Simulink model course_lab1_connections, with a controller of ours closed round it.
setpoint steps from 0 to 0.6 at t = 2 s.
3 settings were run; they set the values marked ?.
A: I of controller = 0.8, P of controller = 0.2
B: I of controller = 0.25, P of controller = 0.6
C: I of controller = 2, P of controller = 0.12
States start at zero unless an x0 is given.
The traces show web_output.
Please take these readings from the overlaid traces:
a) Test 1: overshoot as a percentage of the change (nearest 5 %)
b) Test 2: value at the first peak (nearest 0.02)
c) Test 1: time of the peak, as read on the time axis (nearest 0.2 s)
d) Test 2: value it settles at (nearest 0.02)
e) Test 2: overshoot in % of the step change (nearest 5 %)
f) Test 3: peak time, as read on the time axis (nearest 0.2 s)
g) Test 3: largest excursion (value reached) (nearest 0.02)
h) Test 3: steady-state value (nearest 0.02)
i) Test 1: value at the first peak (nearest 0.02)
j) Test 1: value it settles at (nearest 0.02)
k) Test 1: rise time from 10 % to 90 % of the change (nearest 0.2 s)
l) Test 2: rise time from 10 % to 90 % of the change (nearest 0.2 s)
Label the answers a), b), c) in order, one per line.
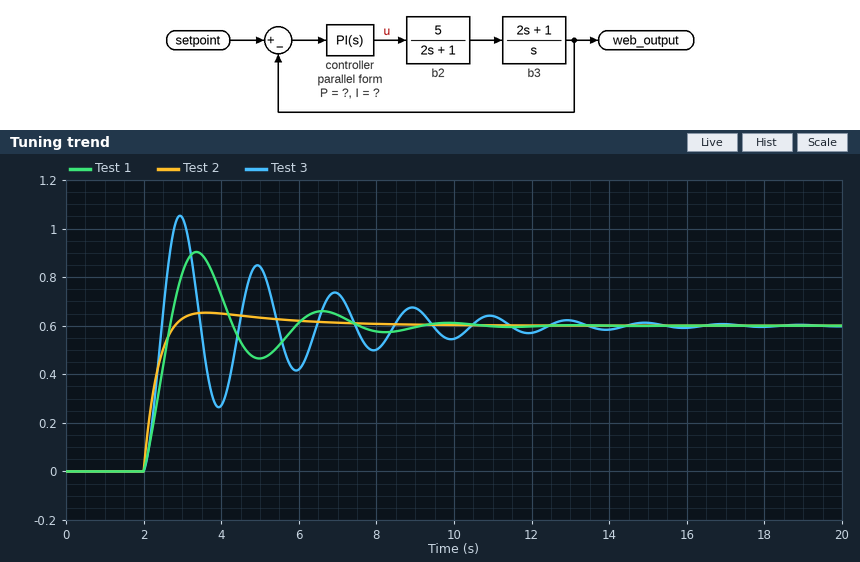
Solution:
a) 50 %
b) 0.66
c) 3.4 s
d) 0.60
e) 10 %
f) 3.0 s
g) 1.06
h) 0.60
i) 0.90
j) 0.60
k) 0.6 s
l) 0.6 s
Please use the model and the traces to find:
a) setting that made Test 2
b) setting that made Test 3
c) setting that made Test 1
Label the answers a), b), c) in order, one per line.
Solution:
a) B
b) C
c) A
